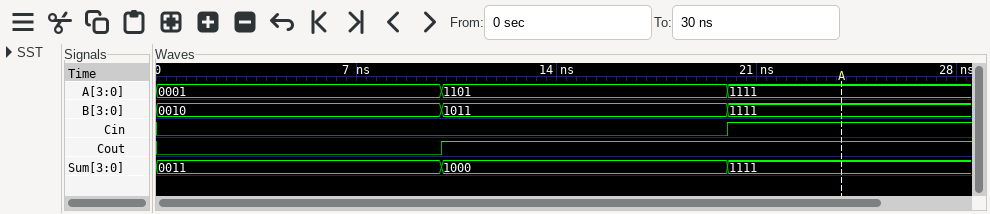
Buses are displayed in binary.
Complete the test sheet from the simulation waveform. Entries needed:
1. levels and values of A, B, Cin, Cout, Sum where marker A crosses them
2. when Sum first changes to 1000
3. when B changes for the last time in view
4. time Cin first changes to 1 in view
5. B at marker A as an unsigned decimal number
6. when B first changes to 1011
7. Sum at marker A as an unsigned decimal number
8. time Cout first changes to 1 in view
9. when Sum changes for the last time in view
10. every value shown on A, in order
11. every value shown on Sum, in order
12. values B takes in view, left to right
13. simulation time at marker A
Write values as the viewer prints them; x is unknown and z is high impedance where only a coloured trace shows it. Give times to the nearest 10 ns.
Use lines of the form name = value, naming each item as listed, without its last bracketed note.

levels and values of A, B, Cin, Cout, Sum where marker A crosses them = A=1111, B=1111, Cin=1, Cout=1, Sum=1111
when Sum first changes to 1000 = 10 ns
when B changes for the last time in view = 20 ns
time Cin first changes to 1 in view = 20 ns
B at marker A as an unsigned decimal number = 15
when B first changes to 1011 = 10 ns
Sum at marker A as an unsigned decimal number = 15
time Cout first changes to 1 in view = 10 ns
when Sum changes for the last time in view = 20 ns
every value shown on A, in order = 0001, 1101, 1111
every value shown on Sum, in order = 0011, 1000, 1111
values B takes in view, left to right = 0010, 1011, 1111
simulation time at marker A = 20 ns
